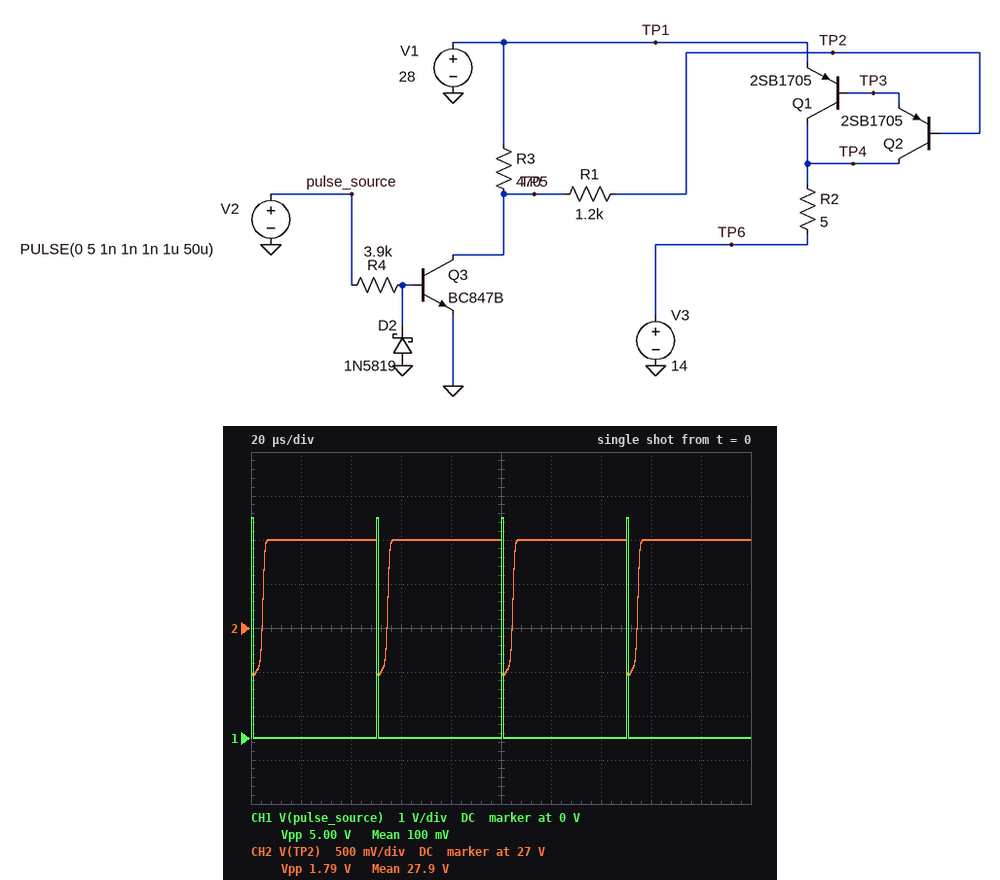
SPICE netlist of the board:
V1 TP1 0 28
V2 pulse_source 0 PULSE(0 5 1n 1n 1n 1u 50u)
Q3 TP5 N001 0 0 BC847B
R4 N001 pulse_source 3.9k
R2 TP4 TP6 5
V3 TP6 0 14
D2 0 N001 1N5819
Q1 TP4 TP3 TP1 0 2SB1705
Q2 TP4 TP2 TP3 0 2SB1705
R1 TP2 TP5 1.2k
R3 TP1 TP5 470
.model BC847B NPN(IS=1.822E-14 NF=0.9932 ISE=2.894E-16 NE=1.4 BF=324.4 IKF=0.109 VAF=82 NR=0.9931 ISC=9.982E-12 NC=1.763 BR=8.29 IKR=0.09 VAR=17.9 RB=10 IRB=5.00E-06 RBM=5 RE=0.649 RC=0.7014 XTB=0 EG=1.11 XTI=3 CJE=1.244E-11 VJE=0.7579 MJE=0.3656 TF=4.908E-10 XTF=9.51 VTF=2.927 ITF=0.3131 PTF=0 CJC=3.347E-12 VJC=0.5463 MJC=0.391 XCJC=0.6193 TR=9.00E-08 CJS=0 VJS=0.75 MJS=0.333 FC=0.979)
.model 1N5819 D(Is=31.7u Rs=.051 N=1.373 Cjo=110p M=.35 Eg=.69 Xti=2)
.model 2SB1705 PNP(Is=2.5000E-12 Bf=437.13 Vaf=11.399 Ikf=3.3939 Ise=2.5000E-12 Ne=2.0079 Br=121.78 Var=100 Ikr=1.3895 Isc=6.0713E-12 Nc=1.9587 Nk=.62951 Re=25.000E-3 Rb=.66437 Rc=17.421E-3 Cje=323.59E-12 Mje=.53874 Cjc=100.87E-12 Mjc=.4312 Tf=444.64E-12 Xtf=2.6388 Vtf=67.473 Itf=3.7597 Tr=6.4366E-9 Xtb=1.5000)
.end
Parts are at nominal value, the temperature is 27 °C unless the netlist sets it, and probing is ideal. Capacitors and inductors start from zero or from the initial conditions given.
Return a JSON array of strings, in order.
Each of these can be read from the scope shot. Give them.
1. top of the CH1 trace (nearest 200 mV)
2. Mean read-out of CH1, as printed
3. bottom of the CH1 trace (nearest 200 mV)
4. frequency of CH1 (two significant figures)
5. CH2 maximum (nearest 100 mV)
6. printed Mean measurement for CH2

["5.0 V", "100 mV", "0 V", "20 kHz", "28.0 V", "27.9 V"]
